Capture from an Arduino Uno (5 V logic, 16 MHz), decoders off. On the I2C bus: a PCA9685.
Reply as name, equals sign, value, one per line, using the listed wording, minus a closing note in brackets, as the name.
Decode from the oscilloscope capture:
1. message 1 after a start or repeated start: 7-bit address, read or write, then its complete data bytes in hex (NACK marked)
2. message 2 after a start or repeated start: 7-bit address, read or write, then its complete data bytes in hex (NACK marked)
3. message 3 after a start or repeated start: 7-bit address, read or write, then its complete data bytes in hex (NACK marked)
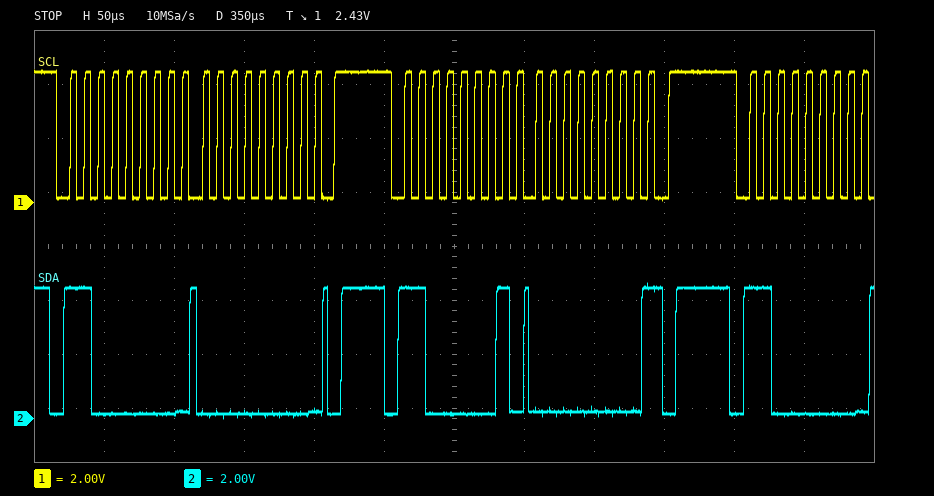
message 1 after a start or repeated start: 7-bit address, read or write, then its complete data bytes in hex = 0x60 write: 00
message 2 after a start or repeated start: 7-bit address, read or write, then its complete data bytes in hex = 0x60 read: 00 NACK
message 3 after a start or repeated start: 7-bit address, read or write, then its complete data bytes in hex = 0x60 write
